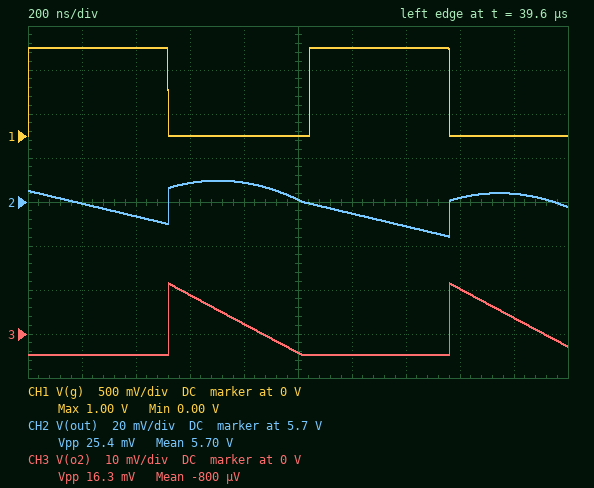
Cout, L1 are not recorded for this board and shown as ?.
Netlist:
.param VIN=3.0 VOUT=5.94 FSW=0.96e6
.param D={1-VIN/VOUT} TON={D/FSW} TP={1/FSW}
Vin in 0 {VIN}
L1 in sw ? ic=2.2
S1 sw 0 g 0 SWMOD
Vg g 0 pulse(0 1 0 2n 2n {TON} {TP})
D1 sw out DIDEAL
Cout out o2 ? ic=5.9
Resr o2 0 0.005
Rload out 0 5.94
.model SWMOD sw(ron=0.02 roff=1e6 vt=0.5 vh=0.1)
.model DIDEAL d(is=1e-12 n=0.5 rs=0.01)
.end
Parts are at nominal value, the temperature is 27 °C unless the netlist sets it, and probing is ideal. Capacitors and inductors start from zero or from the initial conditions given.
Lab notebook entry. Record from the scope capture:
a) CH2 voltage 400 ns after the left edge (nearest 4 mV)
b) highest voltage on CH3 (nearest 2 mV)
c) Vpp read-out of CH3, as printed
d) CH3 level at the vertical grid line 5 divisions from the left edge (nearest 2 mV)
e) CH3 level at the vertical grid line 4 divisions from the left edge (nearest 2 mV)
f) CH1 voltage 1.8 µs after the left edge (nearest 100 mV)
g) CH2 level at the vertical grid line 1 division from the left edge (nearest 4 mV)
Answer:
5.692 V
12 mV
16.3 mV
-4 mV
2 mV
0 V
5.700 V
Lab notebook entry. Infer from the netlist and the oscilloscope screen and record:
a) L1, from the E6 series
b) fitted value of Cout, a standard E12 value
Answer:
470 nH
33 µF
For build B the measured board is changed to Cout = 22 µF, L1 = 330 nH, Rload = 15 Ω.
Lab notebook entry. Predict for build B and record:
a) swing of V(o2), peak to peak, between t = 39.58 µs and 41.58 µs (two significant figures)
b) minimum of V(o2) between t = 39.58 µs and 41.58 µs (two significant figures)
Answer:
23 mV
-2.3 mV
